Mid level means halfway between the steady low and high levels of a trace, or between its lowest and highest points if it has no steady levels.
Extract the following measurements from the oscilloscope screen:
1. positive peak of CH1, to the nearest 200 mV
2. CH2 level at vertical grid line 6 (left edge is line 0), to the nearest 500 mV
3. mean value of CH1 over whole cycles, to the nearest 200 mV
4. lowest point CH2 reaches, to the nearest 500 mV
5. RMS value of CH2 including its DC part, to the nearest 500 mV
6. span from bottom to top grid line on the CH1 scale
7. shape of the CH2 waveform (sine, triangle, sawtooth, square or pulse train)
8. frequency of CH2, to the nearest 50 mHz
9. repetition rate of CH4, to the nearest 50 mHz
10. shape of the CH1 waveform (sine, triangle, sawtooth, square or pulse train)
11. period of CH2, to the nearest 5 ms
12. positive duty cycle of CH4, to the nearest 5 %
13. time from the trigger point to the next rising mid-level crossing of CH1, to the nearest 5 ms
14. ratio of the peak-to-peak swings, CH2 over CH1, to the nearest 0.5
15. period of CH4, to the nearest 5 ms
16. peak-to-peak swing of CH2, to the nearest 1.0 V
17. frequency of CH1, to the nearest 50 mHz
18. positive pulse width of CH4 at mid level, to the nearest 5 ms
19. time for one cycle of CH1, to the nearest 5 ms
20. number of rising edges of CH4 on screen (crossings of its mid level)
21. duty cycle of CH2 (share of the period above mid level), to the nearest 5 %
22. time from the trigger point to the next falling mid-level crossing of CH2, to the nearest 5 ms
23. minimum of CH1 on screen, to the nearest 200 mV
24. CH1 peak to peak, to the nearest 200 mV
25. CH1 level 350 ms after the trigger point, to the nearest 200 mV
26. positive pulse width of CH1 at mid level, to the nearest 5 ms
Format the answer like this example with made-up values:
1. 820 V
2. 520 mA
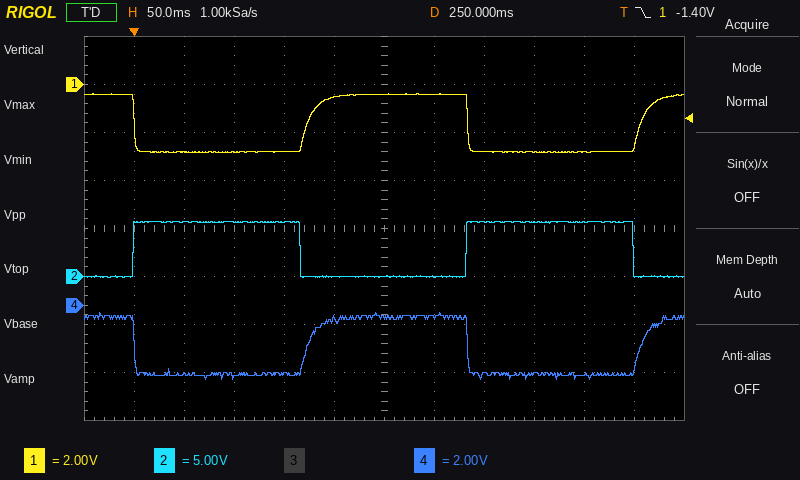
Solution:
1. -400 mV
2. 0.0 V
3. -1.6 V
4. 0.0 V
5. 4.0 V
6. 16 V
7. square
8. 3.00 Hz
9. 3.00 Hz
10. square
11. 335 ms
12. 50 %
13. 175 ms
14. 2.5
15. 335 ms
16. 6.0 V
17. 3.00 Hz
18. 160 ms
19. 335 ms
20. 2
21. 50 %
22. 165 ms
23. -2.8 V
24. 2.4 V
25. -2.8 V
26. 160 ms
